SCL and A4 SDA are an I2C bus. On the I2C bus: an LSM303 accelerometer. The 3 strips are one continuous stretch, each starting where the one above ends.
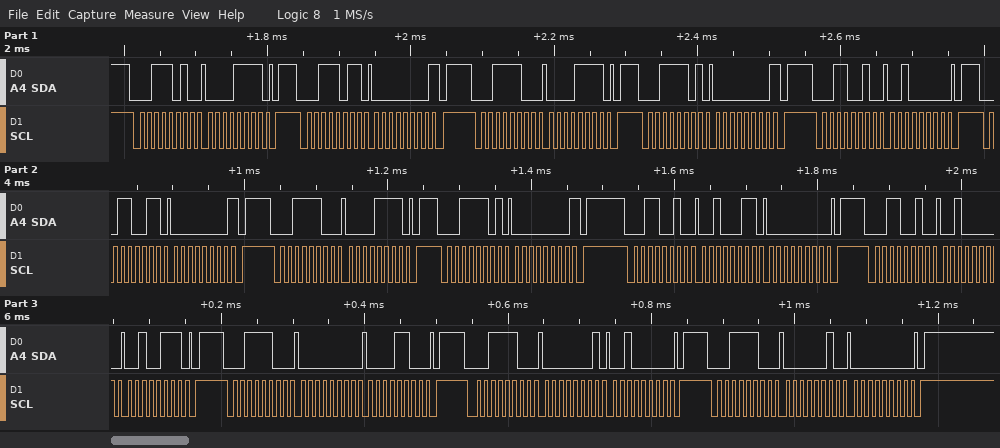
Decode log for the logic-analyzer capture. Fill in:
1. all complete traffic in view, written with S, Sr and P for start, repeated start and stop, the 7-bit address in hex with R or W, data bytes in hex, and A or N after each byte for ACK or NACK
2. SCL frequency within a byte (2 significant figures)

S 1DW A 0F A P S 1DR A 00 N P S 1EW A 0F A P S 1ER A 00 N P S 19W A 20 A P S 19R A 00 N P S 1EW A 0F A P S 1ER A 00 N P S 19W A 23 A 00 A P S 19W A 20 A 27 A P S 1EW A 00 A 0C A P S 1EW A 01 A 20 A P S 1EW A 02 A 00 A P
100 kHz
